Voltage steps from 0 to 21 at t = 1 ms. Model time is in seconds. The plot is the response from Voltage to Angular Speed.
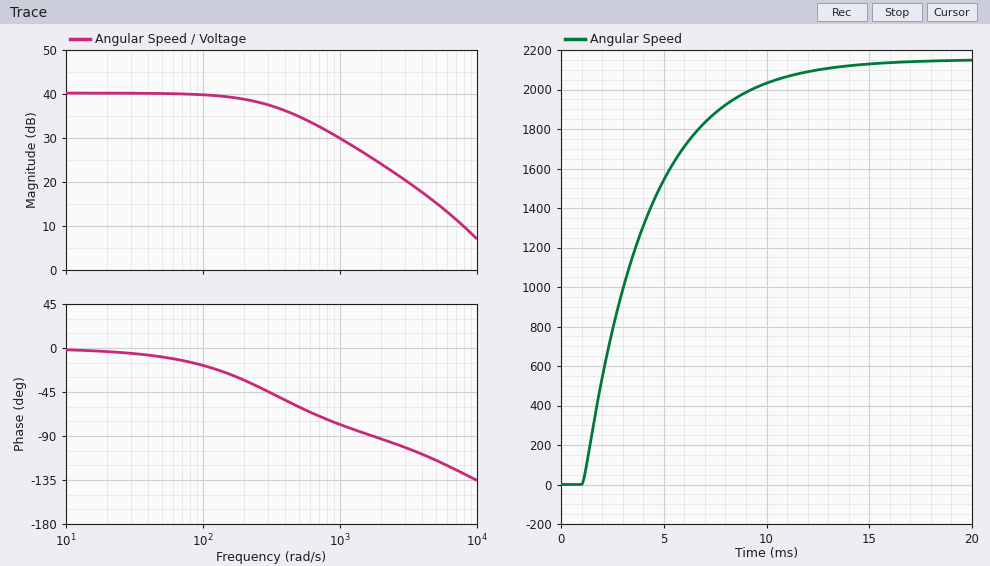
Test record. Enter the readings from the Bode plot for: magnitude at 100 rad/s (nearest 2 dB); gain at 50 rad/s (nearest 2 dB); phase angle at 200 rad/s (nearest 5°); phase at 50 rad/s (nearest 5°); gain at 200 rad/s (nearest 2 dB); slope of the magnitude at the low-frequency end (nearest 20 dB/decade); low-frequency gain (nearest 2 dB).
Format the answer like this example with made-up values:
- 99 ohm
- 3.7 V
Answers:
- 40 dB
- 40 dB
- -35°
- -10°
- 38 dB
- 0 dB/decade
- 40 dB
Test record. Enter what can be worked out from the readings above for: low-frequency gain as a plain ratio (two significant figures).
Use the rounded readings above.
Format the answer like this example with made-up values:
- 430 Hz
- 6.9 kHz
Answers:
- 100
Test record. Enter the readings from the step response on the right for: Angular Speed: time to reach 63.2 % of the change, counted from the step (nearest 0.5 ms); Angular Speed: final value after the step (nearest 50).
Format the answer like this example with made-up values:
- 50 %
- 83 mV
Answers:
- 3.0 ms
- 2150
